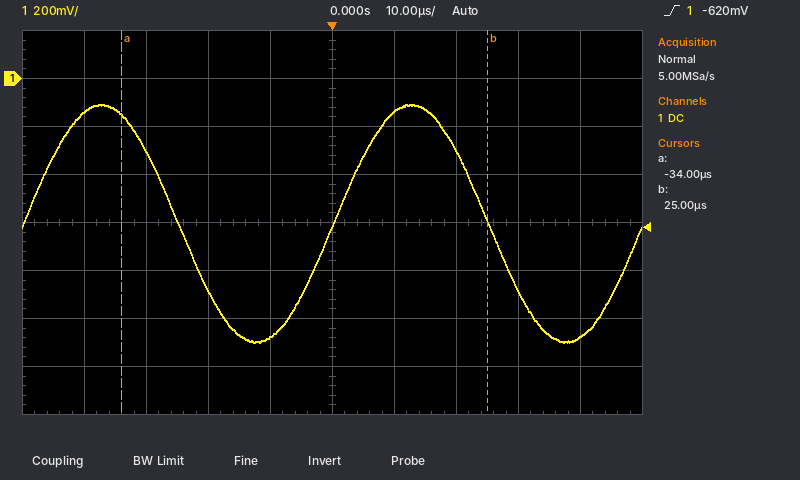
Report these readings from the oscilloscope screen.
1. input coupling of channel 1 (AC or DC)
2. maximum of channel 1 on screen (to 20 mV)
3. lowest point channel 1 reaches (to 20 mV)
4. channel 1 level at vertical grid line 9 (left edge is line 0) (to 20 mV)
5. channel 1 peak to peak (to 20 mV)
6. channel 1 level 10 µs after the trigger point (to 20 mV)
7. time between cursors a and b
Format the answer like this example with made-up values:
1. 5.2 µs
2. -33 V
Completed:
1. DC
2. -100 mV
3. -1.10 V
4. -1.08 V
5. 1.00 V
6. -140 mV
7. 59 µs
